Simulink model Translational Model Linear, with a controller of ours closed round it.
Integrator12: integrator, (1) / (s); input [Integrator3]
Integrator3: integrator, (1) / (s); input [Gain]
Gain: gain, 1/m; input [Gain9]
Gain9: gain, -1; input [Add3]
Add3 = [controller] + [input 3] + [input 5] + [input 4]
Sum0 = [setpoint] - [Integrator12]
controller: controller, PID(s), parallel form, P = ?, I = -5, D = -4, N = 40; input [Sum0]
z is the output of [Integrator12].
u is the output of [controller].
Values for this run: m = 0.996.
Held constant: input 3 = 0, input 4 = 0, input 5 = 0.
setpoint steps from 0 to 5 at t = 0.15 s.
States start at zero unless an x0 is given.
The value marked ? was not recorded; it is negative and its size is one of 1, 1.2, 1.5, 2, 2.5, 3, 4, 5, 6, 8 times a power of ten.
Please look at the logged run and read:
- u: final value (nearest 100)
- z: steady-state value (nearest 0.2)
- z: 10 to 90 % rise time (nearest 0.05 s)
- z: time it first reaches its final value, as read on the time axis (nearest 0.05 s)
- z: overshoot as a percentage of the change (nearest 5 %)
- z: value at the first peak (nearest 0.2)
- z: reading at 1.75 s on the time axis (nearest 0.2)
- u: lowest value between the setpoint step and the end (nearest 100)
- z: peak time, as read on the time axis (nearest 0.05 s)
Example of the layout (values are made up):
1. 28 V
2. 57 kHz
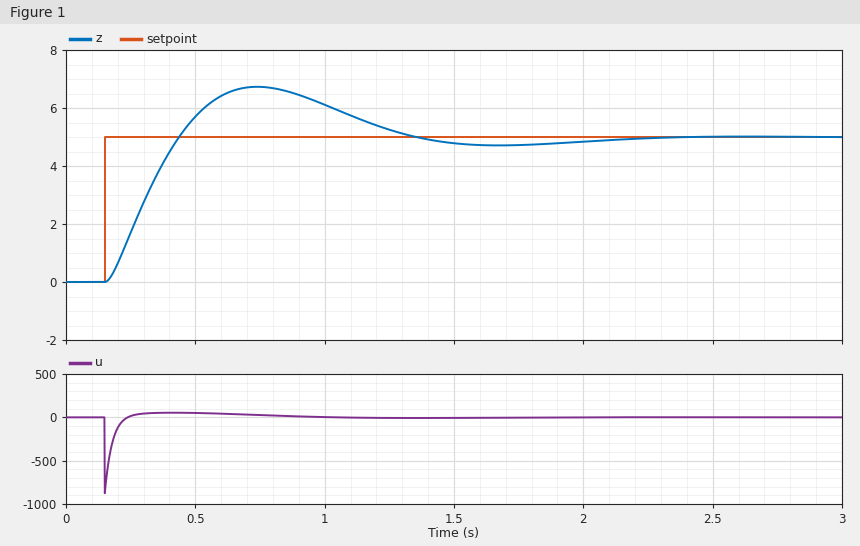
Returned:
1. 0
2. 5.0
3. 0.20 s
4. 0.45 s
5. 35 %
6. 6.8
7. 4.8
8. -900
9. 0.75 s
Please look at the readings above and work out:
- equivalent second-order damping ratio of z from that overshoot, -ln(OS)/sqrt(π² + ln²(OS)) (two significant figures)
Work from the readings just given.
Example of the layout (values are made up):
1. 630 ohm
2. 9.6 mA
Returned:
1. 0.32
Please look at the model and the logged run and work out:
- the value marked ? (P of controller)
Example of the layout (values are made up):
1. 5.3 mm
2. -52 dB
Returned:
1. -15
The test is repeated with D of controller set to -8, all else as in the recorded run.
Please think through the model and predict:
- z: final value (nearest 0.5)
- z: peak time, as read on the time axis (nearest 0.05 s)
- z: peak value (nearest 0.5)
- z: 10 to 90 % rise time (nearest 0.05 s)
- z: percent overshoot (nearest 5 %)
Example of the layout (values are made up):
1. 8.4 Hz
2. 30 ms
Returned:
1. 5.0
2. 0.60 s
3. 6.0
4. 0.15 s
5. 15 %
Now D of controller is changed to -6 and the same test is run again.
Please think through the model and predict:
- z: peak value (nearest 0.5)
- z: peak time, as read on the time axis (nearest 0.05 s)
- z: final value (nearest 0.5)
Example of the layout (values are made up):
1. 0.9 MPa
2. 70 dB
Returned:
1. 6.0
2. 0.65 s
3. 5.0
